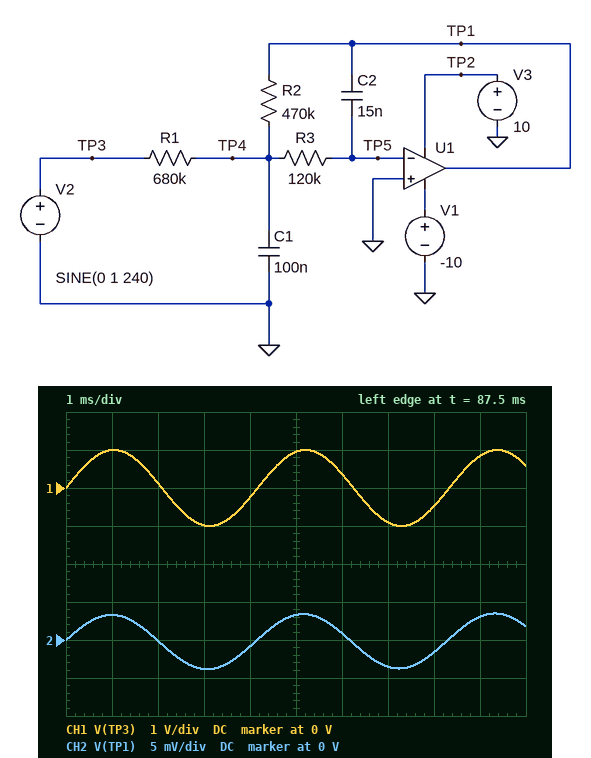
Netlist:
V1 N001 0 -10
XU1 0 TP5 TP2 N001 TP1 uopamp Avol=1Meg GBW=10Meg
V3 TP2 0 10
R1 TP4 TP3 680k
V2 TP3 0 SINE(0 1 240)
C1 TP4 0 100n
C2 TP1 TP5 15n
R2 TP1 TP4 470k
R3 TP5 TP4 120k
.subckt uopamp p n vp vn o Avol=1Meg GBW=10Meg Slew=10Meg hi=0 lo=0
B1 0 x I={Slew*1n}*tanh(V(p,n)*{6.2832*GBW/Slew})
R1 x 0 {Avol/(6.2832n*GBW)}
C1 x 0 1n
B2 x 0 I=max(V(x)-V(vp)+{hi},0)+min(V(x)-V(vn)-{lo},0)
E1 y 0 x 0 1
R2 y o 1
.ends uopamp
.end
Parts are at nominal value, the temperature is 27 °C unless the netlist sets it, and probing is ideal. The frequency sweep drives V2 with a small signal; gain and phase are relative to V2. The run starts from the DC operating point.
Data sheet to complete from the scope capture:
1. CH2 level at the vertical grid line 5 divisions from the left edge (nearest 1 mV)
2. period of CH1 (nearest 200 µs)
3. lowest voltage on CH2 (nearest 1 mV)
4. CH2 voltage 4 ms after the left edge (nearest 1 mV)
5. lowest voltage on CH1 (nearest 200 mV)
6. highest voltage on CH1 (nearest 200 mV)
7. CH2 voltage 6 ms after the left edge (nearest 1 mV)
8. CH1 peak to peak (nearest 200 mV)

3 mV
4.2 ms
-4 mV
-1 mV
-1.0 V
1.0 V
1 mV
2.0 V
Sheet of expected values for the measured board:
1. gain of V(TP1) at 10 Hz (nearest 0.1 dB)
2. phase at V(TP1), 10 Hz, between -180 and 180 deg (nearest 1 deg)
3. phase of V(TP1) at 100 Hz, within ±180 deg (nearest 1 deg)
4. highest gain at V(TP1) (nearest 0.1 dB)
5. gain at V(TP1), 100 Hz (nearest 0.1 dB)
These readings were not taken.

-2.5 dB
136 deg
11 deg
-2.5 dB
-33.6 dB
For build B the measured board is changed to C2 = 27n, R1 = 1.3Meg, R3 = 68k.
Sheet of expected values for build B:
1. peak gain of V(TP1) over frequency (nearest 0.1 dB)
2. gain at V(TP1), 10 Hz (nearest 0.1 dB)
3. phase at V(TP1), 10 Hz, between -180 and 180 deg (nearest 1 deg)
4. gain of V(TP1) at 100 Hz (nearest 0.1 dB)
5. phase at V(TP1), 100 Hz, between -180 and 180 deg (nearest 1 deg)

-8.8 dB
-10.1 dB
125 deg
-39.6 dB
16 deg
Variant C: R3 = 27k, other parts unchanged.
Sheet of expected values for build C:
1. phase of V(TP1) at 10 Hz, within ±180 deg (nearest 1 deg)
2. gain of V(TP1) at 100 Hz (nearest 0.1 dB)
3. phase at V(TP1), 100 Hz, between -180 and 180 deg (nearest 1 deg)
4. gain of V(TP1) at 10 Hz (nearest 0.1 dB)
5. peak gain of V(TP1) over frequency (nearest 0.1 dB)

152 deg
-21.4 dB
37 deg
-3.6 dB
-3.2 dB
